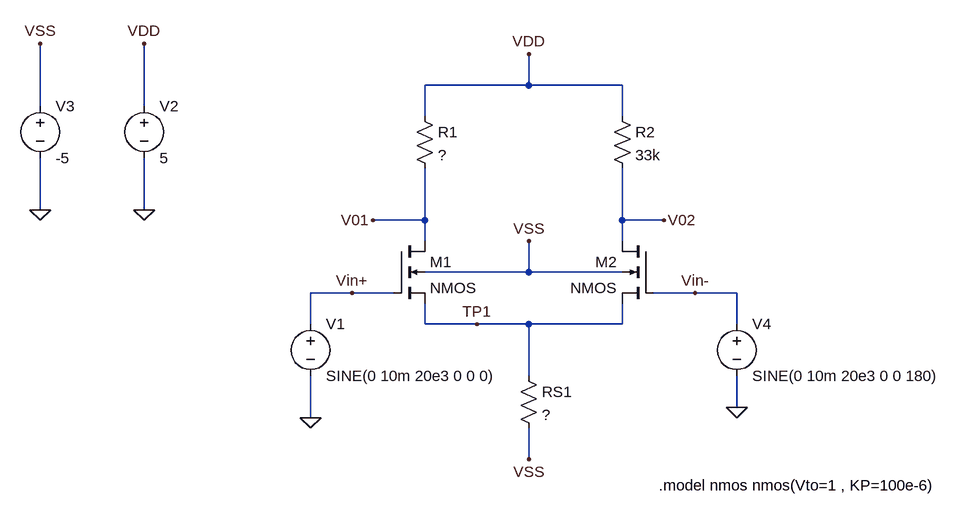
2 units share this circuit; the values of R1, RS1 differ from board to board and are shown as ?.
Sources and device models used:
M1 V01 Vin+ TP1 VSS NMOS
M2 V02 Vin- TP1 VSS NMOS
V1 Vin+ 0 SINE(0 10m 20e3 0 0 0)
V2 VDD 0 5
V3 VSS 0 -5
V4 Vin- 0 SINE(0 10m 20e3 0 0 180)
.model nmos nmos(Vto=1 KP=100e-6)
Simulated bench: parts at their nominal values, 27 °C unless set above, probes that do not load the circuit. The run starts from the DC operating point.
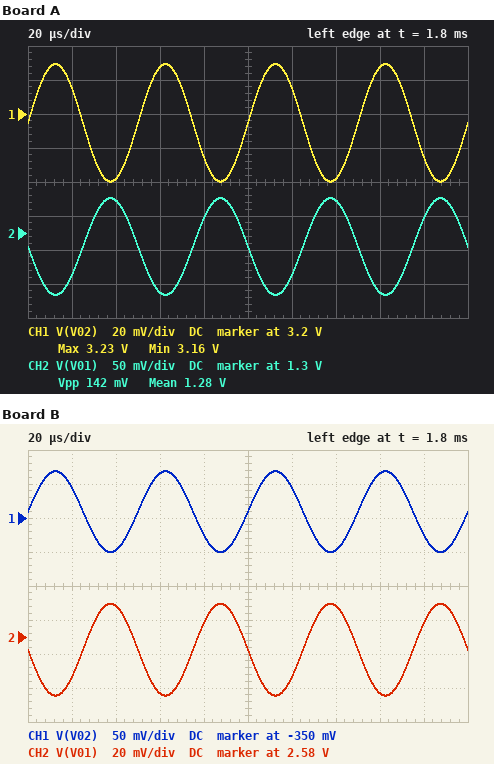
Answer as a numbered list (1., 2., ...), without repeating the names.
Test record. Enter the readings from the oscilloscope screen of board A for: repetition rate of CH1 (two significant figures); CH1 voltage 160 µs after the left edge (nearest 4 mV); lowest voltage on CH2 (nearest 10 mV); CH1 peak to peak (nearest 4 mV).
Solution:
1. 20 kHz
2. 3.228 V
3. 1.21 V
4. 68 mV
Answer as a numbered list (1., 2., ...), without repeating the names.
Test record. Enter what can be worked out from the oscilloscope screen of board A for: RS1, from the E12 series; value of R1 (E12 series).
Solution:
1. 27 kΩ
2. 68 kΩ
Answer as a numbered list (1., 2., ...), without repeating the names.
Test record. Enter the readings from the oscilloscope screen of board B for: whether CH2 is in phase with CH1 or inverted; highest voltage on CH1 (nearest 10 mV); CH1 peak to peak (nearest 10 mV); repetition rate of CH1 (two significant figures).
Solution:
1. inverted
2. -280 mV
3. 120 mV
4. 20 kHz
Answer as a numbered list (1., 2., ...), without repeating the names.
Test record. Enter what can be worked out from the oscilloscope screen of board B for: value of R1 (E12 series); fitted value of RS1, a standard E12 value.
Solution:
1. 15 kΩ
2. 6.8 kΩ
